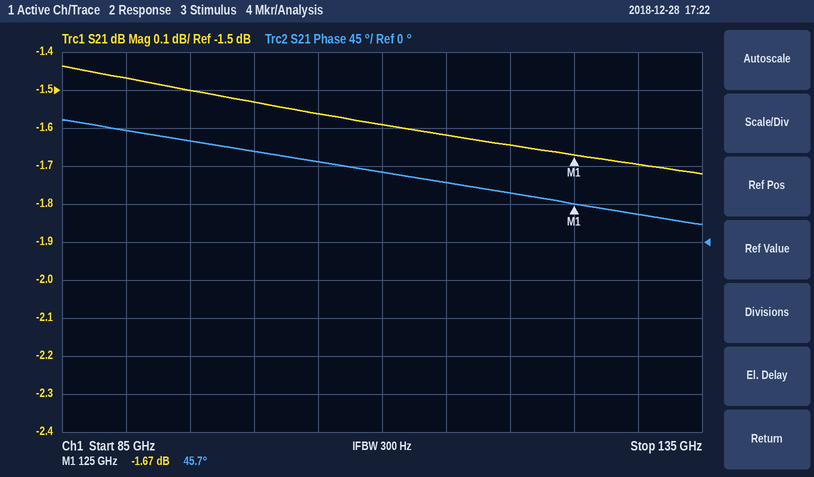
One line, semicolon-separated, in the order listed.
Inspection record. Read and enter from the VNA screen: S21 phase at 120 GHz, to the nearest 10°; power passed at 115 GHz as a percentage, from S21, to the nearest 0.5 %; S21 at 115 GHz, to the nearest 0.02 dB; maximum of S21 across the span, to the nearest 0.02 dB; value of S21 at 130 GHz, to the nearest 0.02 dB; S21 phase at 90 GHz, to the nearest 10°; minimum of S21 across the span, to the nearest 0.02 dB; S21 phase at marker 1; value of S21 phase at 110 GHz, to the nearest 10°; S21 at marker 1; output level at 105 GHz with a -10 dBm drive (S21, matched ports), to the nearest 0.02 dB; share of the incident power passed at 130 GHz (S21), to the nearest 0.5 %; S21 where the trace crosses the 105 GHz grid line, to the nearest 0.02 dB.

60°; 69.0 %; -1.62 dB; -1.44 dB; -1.70 dB; 130°; -1.72 dB; 45.7°; 80°; -1.67 dB; -11.56 dBm; 67.5 %; -1.56 dB
